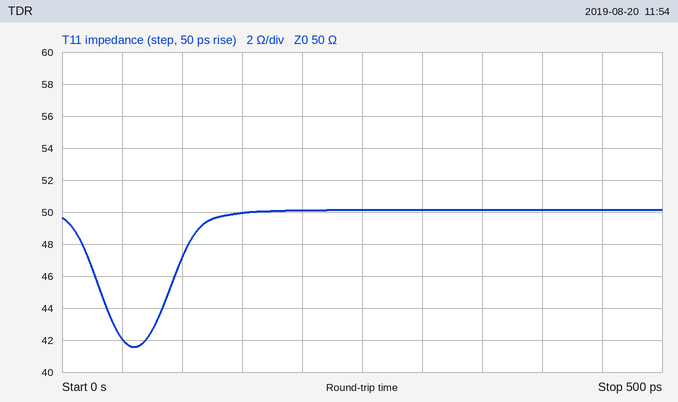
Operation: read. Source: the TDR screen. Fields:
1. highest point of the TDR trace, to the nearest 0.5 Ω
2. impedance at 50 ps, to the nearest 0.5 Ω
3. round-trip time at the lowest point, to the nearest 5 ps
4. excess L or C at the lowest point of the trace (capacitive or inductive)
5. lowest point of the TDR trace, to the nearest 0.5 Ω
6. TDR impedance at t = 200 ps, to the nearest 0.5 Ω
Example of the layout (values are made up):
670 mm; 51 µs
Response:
50.0 Ω; 42.0 Ω; 60 ps; capacitive; 41.5 Ω; 50.0 Ω
